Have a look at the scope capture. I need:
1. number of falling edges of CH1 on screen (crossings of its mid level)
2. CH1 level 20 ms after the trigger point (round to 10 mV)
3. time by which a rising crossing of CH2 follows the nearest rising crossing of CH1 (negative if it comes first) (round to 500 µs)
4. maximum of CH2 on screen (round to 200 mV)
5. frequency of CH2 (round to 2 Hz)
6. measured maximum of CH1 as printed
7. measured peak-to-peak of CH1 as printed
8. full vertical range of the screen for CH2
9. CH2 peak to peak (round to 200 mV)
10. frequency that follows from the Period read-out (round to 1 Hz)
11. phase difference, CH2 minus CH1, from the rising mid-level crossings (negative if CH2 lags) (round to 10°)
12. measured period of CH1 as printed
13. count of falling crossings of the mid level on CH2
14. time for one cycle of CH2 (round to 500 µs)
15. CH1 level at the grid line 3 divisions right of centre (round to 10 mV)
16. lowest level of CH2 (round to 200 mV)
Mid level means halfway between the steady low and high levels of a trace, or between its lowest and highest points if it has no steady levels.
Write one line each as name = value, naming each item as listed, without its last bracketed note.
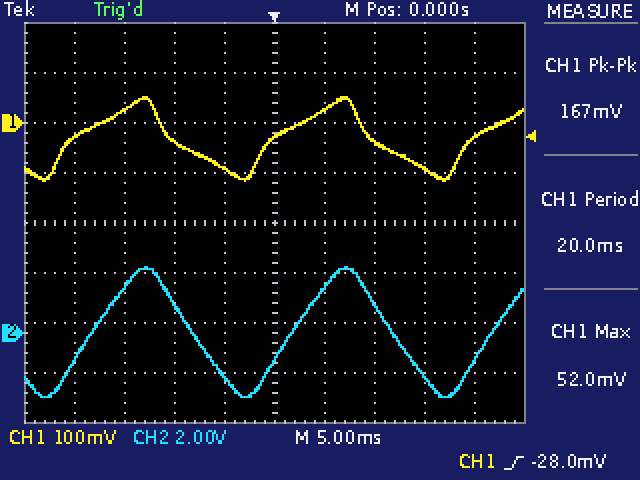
number of falling edges of CH1 on screen = 2
CH1 level 20 ms after the trigger point = -30 mV
time by which a rising crossing of CH2 follows the nearest rising crossing of CH1 (negative if it comes first) = +2.0 ms
maximum of CH2 on screen = 2.6 V
frequency of CH2 = 50 Hz
measured maximum of CH1 as printed = 52.0 mV
measured peak-to-peak of CH1 as printed = 167 mV
full vertical range of the screen for CH2 = 16 V
CH2 peak to peak = 5.2 V
frequency that follows from the Period read-out = 50 Hz
phase difference, CH2 minus CH1, from the rising mid-level crossings (negative if CH2 lags) = -40°
measured period of CH1 as printed = 20.0 ms
count of falling crossings of the mid level on CH2 = 2
time for one cycle of CH2 = 20.0 ms
CH1 level at the grid line 3 divisions right of centre = -90 mV
lowest level of CH2 = -2.6 V
